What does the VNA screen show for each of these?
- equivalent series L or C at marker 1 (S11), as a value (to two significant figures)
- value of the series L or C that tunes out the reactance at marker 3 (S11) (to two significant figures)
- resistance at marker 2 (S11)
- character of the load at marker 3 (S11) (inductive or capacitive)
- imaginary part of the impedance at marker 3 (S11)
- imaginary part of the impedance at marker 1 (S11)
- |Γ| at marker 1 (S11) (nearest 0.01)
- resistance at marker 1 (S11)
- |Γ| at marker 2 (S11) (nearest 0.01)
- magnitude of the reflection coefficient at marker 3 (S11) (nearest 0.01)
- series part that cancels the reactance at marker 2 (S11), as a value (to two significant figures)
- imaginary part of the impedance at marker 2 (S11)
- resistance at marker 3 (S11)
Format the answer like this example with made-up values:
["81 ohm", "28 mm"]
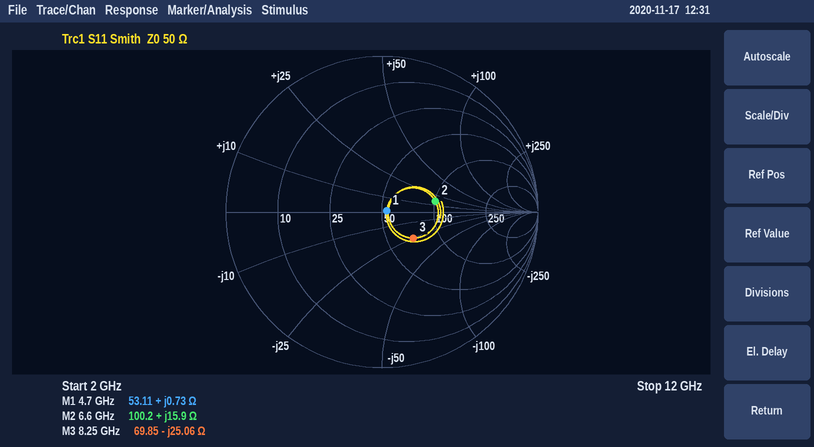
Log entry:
["25 pH", "480 pH", "100.2 Ω", "capacitive", "-25.06 Ω", "+0.73 Ω", "0.03", "53.11 Ω", "0.35", "0.26", "1.5 pF", "+15.9 Ω", "69.85 Ω"]
